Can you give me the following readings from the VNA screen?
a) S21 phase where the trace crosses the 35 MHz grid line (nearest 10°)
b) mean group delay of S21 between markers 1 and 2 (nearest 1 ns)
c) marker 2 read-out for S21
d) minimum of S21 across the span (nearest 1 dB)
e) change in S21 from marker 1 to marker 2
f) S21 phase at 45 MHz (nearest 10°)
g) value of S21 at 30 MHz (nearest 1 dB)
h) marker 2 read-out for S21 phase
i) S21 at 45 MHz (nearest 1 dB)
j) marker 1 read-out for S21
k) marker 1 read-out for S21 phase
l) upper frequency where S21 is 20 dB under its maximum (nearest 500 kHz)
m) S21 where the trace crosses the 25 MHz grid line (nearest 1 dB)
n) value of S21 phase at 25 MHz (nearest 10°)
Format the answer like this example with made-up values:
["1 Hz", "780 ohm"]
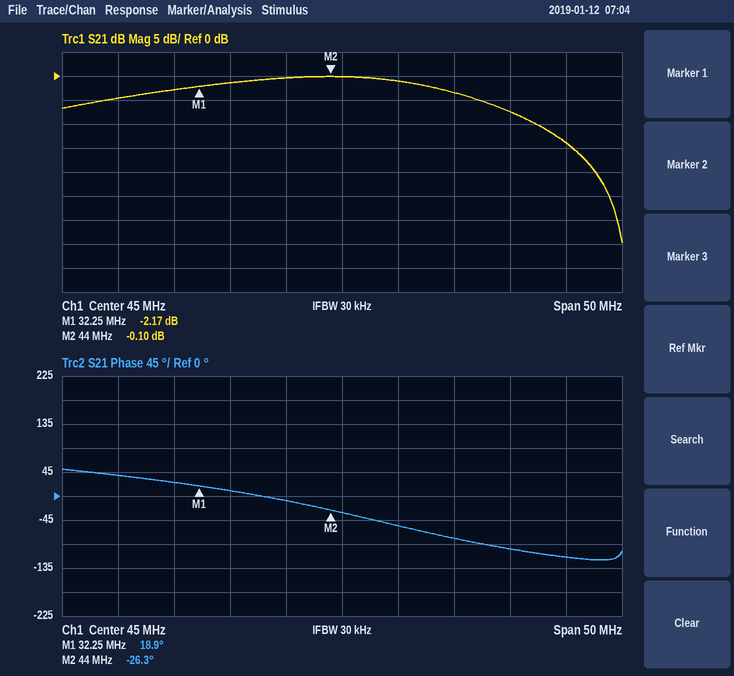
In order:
["10°", "11 ns", "-0.10 dB", "-35 dB", "2.07 dB", "-30°", "-3 dB", "-26.3°", "0 dB", "-2.17 dB", "18.9°", "67.5 MHz", "-5 dB", "40°"]
